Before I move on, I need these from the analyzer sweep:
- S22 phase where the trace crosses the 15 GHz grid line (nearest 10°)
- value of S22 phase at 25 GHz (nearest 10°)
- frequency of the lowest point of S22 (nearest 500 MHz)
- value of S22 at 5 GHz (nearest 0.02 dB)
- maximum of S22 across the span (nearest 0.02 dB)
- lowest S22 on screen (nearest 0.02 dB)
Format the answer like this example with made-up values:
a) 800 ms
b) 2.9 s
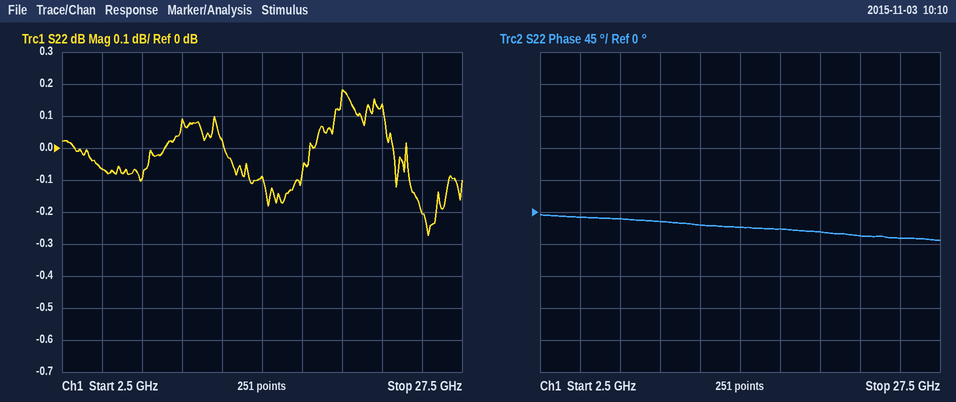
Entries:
a) -20°
b) -40°
c) 25.5 GHz
d) -0.06 dB
e) 0.18 dB
f) -0.28 dB
